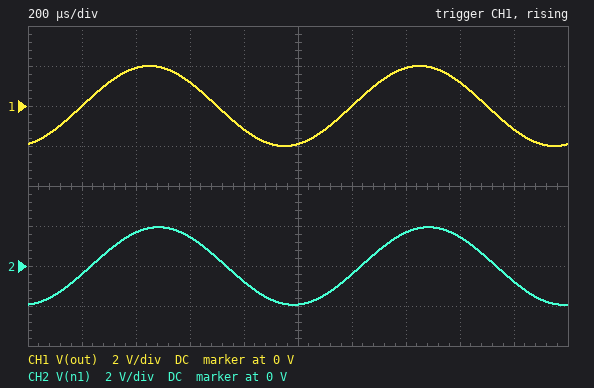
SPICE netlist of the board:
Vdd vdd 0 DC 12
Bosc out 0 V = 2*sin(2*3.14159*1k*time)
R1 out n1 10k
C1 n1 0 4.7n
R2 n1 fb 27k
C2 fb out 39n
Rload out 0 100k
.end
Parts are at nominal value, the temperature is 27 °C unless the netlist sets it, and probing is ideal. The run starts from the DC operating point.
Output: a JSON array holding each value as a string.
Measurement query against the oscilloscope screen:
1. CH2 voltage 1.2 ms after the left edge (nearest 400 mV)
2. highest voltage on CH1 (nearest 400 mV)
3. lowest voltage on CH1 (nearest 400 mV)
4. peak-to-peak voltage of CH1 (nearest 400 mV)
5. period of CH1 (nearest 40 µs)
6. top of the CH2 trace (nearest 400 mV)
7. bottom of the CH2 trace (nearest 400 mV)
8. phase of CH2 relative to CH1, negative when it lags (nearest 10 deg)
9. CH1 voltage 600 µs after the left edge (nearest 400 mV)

["-400 mV", "2.0 V", "-2.0 V", "4.0 V", "1.00 ms", "2.0 V", "-2.0 V", "-10 deg", "1.2 V"]
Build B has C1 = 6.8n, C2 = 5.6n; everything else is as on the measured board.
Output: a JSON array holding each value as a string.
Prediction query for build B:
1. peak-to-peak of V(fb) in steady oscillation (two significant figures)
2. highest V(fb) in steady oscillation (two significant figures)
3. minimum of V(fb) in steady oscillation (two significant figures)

["3.1 V", "1.6 V", "-1.6 V"]
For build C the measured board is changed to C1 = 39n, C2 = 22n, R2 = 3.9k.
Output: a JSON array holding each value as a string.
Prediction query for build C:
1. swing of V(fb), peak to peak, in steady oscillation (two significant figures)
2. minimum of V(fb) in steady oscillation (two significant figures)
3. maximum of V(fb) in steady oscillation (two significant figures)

["1.8 V", "-890 mV", "890 mV"]
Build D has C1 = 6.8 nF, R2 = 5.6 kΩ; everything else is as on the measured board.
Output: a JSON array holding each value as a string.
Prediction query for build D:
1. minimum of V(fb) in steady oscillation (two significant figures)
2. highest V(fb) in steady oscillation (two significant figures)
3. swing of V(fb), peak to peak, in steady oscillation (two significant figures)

["-1.8 V", "1.8 V", "3.6 V"]
